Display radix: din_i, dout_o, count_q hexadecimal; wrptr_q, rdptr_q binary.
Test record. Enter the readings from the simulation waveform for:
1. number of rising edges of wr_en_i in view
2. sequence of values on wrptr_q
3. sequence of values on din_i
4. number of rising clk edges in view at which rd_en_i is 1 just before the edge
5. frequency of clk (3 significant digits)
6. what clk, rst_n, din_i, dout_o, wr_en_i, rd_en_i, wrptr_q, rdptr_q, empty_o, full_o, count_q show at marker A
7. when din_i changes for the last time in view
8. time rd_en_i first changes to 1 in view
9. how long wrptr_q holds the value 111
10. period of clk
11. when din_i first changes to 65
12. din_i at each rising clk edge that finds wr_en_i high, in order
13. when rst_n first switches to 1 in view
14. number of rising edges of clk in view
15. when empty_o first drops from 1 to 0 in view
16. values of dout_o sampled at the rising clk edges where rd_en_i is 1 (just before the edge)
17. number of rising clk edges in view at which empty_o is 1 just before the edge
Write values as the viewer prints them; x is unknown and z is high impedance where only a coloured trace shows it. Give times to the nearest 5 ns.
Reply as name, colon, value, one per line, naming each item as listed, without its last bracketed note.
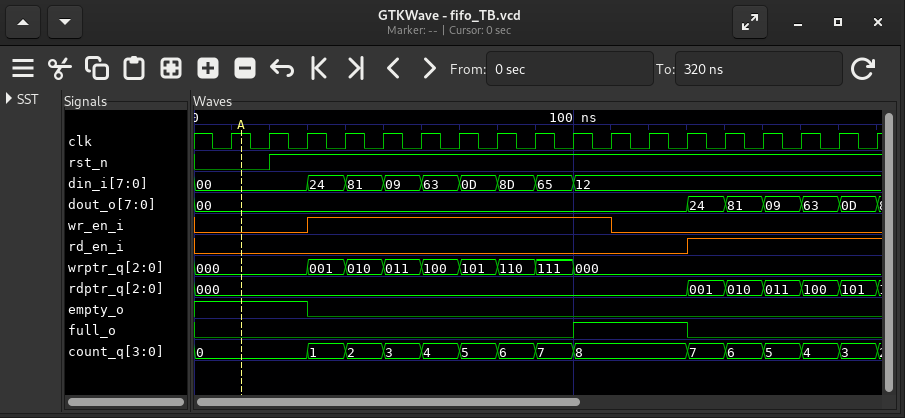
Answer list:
number of rising edges of wr_en_i in view: 1
sequence of values on wrptr_q: 000, 001, 010, 011, 100, 101, 110, 111, 000
sequence of values on din_i: 00, 24, 81, 09, 63, 0D, 8D, 65, 12
number of rising clk edges in view at which rd_en_i is 1 just before the edge: 5
frequency of clk: 100 MHz
what clk, rst_n, din_i, dout_o, wr_en_i, rd_en_i, wrptr_q, rdptr_q, empty_o, full_o, count_q show at marker A: clk=1, rst_n=0, din_i=00, dout_o=00, wr_en_i=0, rd_en_i=0, wrptr_q=000, rdptr_q=000, empty_o=1, full_o=0, count_q=0
when din_i changes for the last time in view: 100 ns
time rd_en_i first changes to 1 in view: 130 ns
how long wrptr_q holds the value 111: 10 ns
period of clk: 10 ns
when din_i first changes to 65: 90 ns
din_i at each rising clk edge that finds wr_en_i high, in order: 24, 81, 09, 63, 0D, 8D, 65, 12
when rst_n first switches to 1 in view: 20 ns
number of rising edges of clk in view: 18
when empty_o first drops from 1 to 0 in view: 30 ns
values of dout_o sampled at the rising clk edges where rd_en_i is 1: 24, 81, 09, 63, 0D
number of rising clk edges in view at which empty_o is 1 just before the edge: 3
